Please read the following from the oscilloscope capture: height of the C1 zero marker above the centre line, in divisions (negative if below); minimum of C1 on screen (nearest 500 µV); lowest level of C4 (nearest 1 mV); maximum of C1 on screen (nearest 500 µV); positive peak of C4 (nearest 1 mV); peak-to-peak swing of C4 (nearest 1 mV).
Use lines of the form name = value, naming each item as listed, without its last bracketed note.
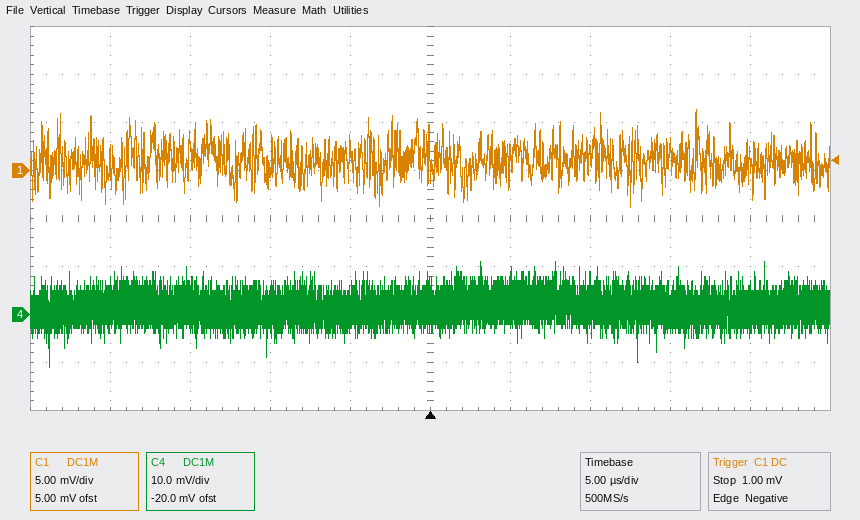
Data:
height of the C1 zero marker above the centre line, in divisions = +1.0 div
minimum of C1 on screen = -4.0 mV
lowest level of C4 = -11 mV
maximum of C1 on screen = 6.5 mV
positive peak of C4 = 11 mV
peak-to-peak swing of C4 = 22 mV
